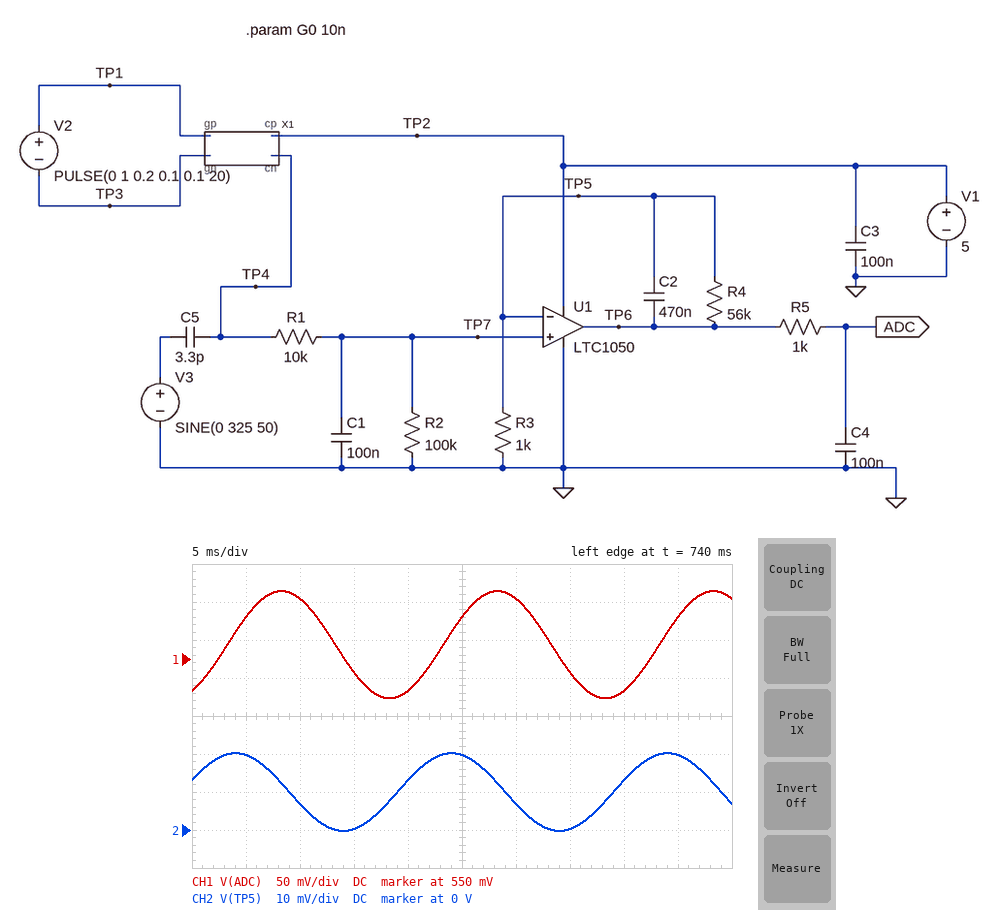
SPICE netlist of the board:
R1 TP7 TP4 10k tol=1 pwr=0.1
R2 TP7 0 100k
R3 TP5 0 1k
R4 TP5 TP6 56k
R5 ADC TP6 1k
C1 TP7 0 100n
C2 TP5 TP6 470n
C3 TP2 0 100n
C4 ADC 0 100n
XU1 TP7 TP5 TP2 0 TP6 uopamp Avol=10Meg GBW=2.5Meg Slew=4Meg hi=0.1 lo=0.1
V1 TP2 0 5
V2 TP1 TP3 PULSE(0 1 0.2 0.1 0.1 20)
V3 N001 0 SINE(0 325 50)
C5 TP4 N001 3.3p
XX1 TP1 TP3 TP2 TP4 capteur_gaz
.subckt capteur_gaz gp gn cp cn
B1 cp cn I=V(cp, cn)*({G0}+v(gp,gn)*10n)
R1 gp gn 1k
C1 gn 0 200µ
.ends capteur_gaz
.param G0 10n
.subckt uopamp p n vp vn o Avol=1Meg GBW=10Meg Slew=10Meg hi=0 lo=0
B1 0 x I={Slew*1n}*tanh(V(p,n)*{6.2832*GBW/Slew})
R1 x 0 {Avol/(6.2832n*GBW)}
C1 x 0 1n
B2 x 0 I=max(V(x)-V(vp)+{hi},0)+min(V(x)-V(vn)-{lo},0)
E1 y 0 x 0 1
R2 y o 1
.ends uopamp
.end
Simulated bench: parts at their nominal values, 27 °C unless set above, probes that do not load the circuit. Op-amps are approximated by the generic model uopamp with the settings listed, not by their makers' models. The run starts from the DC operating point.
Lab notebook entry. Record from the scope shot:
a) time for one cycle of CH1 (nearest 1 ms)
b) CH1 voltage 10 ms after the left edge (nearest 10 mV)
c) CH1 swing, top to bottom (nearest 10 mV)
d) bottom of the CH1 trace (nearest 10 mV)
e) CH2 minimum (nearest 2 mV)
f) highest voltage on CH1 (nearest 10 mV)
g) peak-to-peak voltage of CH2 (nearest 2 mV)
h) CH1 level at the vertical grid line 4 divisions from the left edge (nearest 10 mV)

20 ms
630 mV
140 mV
500 mV
0 V
640 mV
20 mV
510 mV
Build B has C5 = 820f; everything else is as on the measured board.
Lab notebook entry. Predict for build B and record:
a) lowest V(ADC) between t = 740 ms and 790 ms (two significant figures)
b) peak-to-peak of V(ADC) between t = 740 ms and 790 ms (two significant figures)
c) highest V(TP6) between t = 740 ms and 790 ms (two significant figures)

550 mV
35 mV
590 mV
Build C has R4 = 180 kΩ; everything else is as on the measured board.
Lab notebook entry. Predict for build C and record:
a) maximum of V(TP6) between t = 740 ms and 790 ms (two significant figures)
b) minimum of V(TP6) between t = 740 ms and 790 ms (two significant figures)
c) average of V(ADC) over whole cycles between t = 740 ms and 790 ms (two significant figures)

1.9 V
1.7 V
1.8 V
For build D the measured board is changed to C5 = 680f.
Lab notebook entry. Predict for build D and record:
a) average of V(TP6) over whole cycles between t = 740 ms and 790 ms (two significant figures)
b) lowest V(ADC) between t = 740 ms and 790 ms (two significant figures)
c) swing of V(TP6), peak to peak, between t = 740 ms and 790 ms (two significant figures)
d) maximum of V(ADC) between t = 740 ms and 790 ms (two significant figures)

570 mV
550 mV
29 mV
580 mV
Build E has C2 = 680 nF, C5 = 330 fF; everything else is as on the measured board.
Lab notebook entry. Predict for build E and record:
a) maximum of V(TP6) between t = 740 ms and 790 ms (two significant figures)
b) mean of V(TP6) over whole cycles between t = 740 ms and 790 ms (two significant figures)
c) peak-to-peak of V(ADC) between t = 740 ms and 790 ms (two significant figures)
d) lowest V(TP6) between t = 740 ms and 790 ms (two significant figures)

570 mV
570 mV
9.9 mV
560 mV
